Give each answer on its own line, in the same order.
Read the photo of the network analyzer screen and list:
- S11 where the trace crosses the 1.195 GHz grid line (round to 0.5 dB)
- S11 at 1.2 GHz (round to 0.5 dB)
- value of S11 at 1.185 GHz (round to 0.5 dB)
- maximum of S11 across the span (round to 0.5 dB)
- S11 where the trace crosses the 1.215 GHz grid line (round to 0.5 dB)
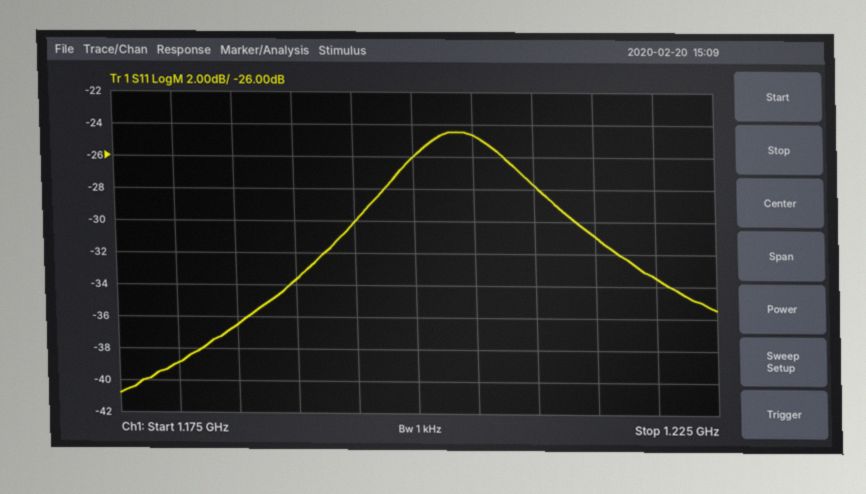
-30.0 dB
-26.0 dB
-36.5 dB
-24.5 dB
-31.0 dB
